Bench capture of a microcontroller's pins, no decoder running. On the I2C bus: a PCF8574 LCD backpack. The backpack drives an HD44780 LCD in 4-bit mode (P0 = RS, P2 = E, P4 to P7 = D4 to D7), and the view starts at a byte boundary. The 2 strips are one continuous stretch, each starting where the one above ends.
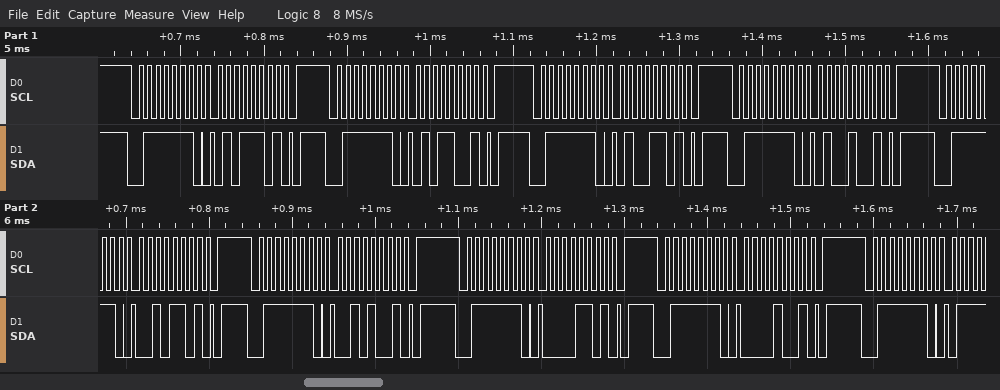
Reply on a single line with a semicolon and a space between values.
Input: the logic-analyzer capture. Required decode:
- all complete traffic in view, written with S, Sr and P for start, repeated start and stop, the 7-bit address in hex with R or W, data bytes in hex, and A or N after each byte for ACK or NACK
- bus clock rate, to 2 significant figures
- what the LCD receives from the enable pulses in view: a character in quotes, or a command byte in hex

S 3FW A 5D A P S 3FW A 59 A P S 3FW A 4D A P S 3FW A 49 A P S 3FW A 2D A P S 3FW A 29 A P S 3FW A 0D A P S 3FW A 09 A P S 3FW A; 100 kHz; 'T' ' '
